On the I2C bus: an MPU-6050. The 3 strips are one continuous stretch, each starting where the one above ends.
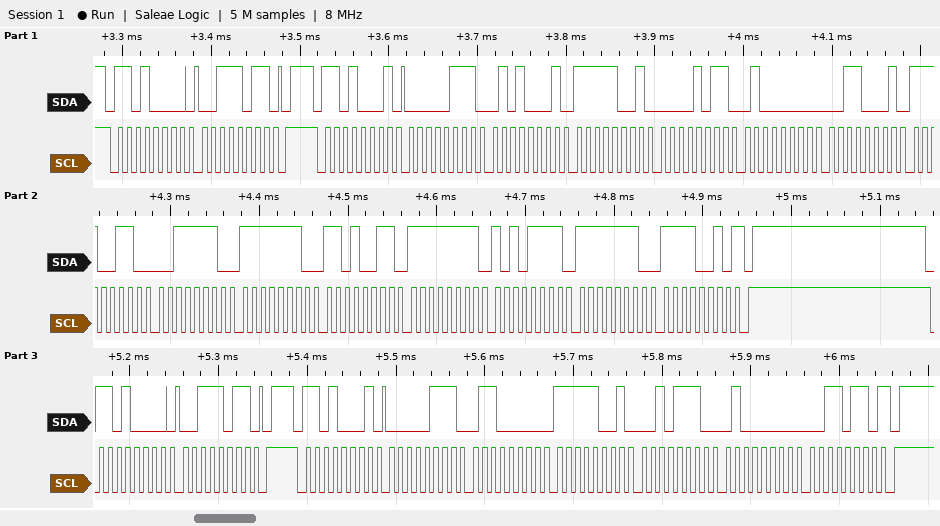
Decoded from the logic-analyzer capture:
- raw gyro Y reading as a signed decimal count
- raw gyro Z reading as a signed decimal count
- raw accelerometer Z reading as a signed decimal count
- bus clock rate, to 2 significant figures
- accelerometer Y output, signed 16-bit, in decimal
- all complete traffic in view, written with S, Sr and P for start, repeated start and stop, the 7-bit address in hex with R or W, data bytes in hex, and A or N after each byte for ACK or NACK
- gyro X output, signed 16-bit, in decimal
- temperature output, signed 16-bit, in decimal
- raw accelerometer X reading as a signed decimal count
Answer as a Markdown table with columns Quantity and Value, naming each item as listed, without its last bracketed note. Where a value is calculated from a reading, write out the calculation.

| Quantity | Value |
|---|---|
| raw gyro Y reading as a signed decimal count | 0xFFAF = -81 |
| raw gyro Z reading as a signed decimal count | 0xFEF2 = -270 |
| raw accelerometer Z reading as a signed decimal count | 0x4031 = 16433 |
| bus clock rate, to 2 significant figures | 100 kHz |
| accelerometer Y output, signed 16-bit, in decimal | 0xF90B = -1781 |
| all complete traffic in view, written with S, Sr and P for start, repeated start and stop, the 7-bit address in hex with R or W, data bytes in hex, and A or N after each byte for ACK or NACK | S 68W A 3B A P S 68R A 07 A 51 A F9 A 0B A 40 A 31 A E6 A 3E A FE A D3 A FF A AF A FE A F2 N P S 68W A 3B A P S 68R A 07 A 60 A F9 A 2E A 40 A 36 N P |
| gyro X output, signed 16-bit, in decimal | 0xFED3 = -301 |
| temperature output, signed 16-bit, in decimal | 0xE63E = -6594 |
| raw accelerometer X reading as a signed decimal count | 0x0751 = 1873 |
